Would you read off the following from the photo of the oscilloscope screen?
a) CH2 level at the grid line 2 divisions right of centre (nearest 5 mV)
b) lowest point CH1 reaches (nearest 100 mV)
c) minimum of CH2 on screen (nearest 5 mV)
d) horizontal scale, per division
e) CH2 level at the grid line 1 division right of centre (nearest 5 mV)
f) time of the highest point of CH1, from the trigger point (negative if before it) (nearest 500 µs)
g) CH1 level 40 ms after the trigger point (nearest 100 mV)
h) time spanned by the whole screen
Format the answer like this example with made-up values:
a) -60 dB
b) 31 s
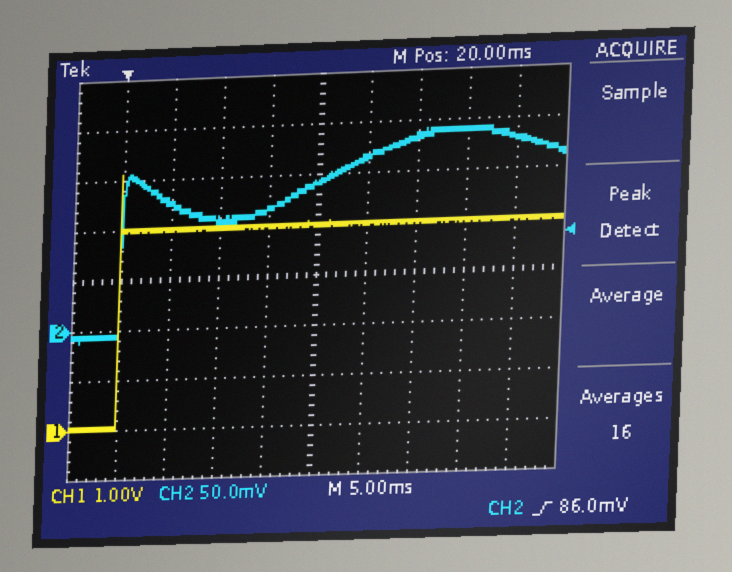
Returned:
a) 185 mV
b) 0.0 V
c) -10 mV
d) 5 ms
e) 165 mV
f) 0.0 ms
g) 4.0 V
h) 50 ms
